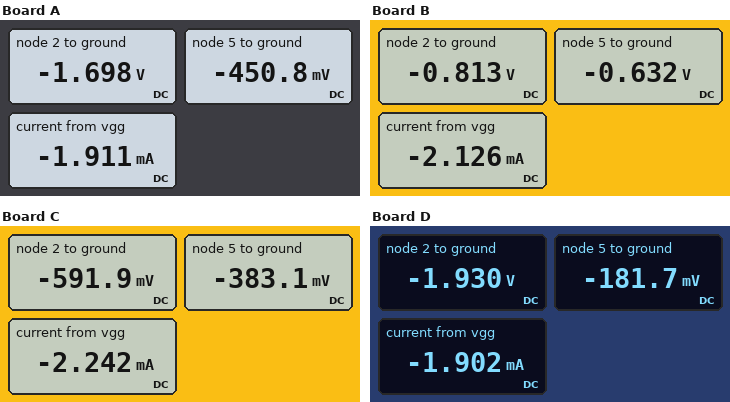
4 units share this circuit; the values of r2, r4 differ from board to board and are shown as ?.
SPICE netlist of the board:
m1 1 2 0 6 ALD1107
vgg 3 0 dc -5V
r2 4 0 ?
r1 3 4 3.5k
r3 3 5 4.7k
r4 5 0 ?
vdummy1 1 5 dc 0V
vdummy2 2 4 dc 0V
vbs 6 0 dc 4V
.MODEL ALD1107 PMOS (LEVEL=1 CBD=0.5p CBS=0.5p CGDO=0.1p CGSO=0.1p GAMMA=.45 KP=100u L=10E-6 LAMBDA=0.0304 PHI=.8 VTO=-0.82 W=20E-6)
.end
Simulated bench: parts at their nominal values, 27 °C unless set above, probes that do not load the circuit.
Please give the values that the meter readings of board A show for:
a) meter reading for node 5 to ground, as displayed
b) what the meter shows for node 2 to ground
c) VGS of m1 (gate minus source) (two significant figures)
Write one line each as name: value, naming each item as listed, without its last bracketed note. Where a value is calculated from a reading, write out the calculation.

meter reading for node 5 to ground, as displayed: -450.8 mV
what the meter shows for node 2 to ground: -1.698 V
VGS of m1 (gate minus source): -1.698 V = -1.7 V
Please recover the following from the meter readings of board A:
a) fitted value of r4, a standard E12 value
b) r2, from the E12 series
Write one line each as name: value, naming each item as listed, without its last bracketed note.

fitted value of r4, a standard E12 value: 470 Ω
r2, from the E12 series: 1.8 kΩ
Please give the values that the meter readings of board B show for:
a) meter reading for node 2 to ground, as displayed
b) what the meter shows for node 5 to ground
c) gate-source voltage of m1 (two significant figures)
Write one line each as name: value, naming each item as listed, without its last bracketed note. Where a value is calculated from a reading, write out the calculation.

meter reading for node 2 to ground, as displayed: -0.813 V
what the meter shows for node 5 to ground: -0.632 V
gate-source voltage of m1: -813 mV = -810 mV
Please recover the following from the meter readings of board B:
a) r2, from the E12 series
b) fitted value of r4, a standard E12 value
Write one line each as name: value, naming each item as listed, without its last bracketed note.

r2, from the E12 series: 680 Ω
fitted value of r4, a standard E12 value: 680 Ω
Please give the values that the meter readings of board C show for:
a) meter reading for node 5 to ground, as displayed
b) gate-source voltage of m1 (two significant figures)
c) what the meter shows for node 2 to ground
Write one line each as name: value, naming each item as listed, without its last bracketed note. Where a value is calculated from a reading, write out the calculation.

meter reading for node 5 to ground, as displayed: -383.1 mV
gate-source voltage of m1: -591.9 mV = -590 mV
what the meter shows for node 2 to ground: -591.9 mV
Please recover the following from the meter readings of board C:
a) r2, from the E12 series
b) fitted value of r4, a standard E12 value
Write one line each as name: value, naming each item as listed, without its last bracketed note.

r2, from the E12 series: 470 Ω
fitted value of r4, a standard E12 value: 390 Ω
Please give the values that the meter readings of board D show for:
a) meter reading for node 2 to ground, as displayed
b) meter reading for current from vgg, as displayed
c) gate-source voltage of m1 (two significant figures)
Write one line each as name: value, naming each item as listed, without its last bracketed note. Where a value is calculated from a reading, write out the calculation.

meter reading for node 2 to ground, as displayed: -1.930 V
meter reading for current from vgg, as displayed: -1.902 mA
gate-source voltage of m1: -1.93 V = -1.9 V
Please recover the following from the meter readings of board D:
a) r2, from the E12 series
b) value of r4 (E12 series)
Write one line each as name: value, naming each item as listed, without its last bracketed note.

r2, from the E12 series: 2.2 kΩ
value of r4: 180 Ω
